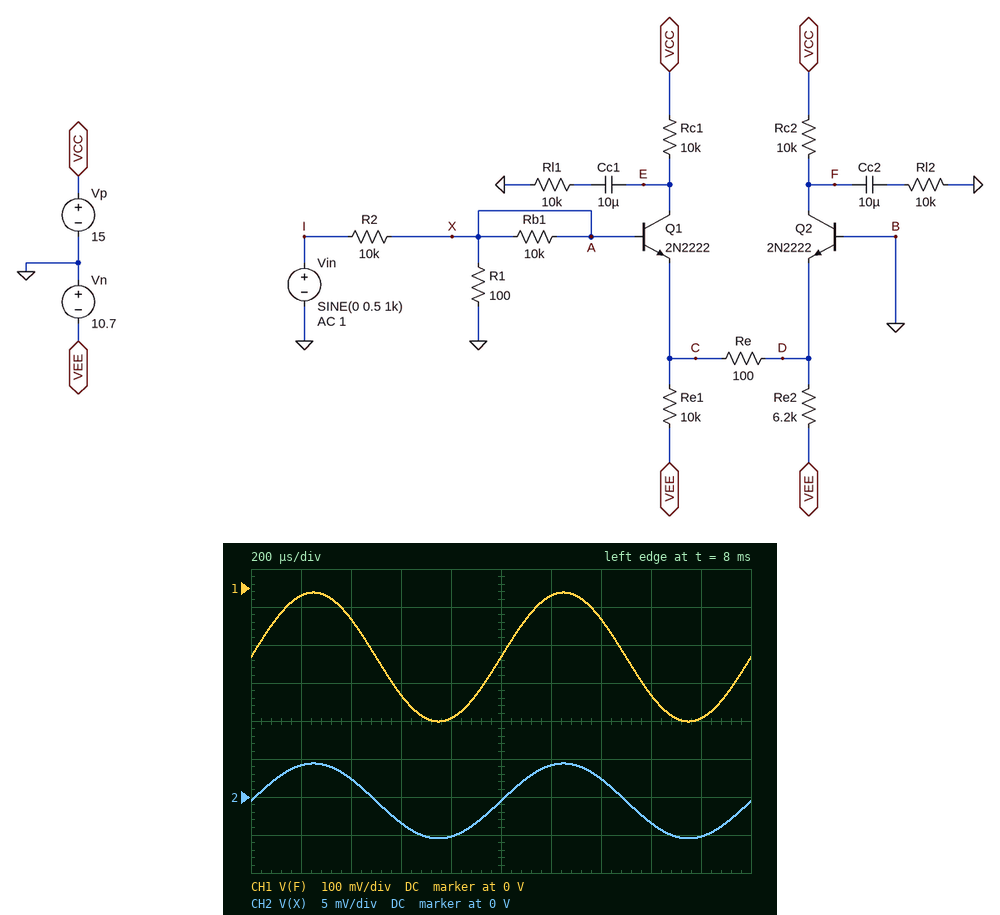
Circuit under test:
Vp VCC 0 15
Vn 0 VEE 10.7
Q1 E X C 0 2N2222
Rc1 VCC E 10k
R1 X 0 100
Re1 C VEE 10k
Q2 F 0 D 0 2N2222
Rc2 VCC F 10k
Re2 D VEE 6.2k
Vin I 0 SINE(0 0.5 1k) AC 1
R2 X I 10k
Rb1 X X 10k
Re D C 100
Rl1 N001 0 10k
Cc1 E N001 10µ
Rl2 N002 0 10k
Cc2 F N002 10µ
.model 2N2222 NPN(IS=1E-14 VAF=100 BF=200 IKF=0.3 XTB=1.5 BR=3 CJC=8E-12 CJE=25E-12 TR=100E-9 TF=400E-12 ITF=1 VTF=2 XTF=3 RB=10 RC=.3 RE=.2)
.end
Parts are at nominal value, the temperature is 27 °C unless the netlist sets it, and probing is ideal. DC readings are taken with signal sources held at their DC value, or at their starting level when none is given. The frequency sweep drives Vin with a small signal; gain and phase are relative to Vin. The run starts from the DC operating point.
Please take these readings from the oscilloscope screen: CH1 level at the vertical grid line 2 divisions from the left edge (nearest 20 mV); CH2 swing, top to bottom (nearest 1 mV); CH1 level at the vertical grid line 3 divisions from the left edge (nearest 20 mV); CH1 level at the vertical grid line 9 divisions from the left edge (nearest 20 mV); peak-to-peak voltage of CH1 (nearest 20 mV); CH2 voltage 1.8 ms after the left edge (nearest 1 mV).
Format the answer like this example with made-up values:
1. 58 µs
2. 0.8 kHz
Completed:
1. -80 mV
2. 10 mV
3. -280 mV
4. -340 mV
5. 340 mV
6. -5 mV
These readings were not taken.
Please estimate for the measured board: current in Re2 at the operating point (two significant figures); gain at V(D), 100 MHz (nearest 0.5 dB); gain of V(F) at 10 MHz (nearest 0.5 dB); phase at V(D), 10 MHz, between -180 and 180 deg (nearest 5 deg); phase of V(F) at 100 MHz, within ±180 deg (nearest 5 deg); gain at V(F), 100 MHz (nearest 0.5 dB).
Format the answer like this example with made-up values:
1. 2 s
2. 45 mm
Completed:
1. 1.6 mA
2. -61.0 dB
3. -23.0 dB
4. -10 deg
5. -115 deg
6. -45.0 dB
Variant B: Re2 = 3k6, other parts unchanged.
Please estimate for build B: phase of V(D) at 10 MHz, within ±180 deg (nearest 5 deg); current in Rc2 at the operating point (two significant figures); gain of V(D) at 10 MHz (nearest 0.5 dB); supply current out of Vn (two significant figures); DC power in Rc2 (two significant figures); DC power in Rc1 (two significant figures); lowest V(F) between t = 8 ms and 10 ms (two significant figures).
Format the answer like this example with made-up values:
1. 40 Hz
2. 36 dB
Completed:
1. -15 deg
2. 1.6 mA
3. -63.5 dB
4. 3.8 mA
5. 25 mW
6. 19 mW
7. -690 mV
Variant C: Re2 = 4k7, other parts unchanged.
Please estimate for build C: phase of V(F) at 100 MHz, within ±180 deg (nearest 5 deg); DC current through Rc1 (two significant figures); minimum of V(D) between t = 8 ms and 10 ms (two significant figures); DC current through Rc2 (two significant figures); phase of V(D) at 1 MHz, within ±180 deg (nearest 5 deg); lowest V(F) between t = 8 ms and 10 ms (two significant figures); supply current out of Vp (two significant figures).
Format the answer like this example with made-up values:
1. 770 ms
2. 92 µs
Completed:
1. 0 deg
2. 1.2 mA
3. -690 mV
4. 1.6 mA
5. -25 deg
6. -660 mV
7. 2.8 mA
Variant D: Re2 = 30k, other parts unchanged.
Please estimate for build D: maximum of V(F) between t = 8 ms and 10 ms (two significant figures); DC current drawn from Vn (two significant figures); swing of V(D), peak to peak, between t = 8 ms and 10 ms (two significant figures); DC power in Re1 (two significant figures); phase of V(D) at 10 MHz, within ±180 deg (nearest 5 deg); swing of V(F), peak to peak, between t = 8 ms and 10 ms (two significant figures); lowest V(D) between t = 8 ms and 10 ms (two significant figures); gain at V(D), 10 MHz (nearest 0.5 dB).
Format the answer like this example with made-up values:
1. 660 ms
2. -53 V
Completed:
1. 10 V
2. 1.3 mA
3. 2.9 mV
4. 10 mW
5. -15 deg
6. 260 mV
7. -640 mV
8. -53.5 dB
